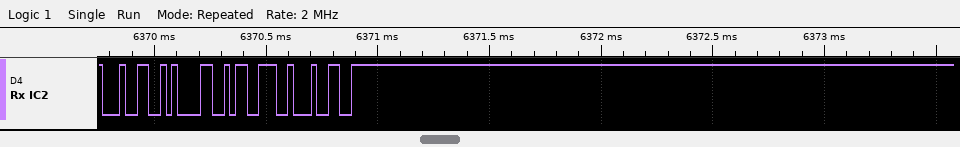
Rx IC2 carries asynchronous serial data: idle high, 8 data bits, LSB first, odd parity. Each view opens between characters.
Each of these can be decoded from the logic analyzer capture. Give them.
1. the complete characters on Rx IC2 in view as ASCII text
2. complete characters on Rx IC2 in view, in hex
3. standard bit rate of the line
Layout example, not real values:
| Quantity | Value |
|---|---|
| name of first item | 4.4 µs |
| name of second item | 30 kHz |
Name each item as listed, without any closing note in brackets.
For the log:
| Quantity | Value |
|---|---|
| the complete characters on Rx IC2 in view as ASCII text | "dasd" |
| complete characters on Rx IC2 in view, in hex | 64, 61, 73, 64 |
| standard bit rate of the line | 38400 baud |
